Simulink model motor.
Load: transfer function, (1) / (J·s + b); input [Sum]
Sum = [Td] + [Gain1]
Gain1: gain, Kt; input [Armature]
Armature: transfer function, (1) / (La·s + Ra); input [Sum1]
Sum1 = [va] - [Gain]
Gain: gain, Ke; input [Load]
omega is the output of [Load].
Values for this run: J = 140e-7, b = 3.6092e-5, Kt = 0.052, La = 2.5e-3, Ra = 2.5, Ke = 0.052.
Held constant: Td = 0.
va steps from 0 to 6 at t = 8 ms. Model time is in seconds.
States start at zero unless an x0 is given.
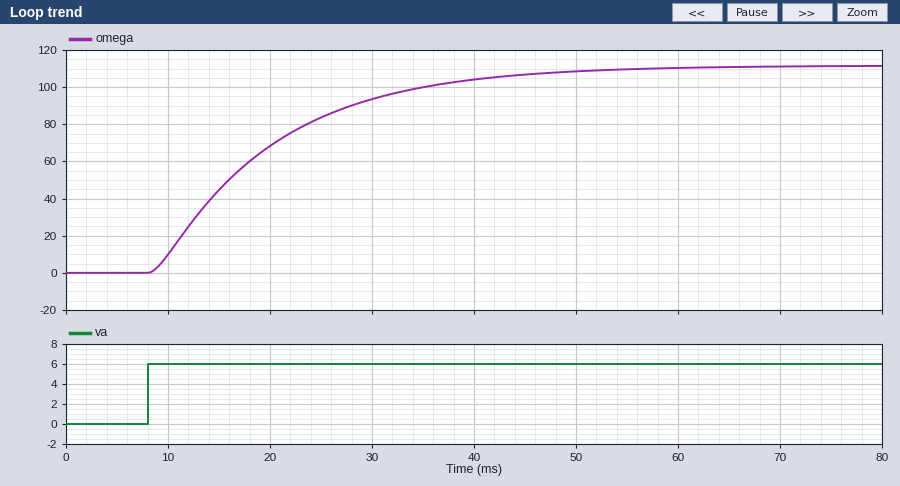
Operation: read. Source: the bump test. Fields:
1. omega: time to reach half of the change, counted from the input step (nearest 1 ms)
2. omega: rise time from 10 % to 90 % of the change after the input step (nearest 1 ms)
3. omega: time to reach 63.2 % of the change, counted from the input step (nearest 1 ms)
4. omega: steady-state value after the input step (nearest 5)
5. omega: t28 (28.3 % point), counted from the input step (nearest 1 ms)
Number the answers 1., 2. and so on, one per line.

1. 9 ms
2. 25 ms
3. 13 ms
4. 110
5. 5 ms
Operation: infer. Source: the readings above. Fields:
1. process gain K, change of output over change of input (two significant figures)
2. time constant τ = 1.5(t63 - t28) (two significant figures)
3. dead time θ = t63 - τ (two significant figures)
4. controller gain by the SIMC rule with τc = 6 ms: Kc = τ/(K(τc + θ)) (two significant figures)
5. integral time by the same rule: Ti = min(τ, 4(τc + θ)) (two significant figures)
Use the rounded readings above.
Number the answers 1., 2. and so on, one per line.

1. 18
2. 12 ms
3. 1.0 ms
4. 0.095
5. 12 ms
